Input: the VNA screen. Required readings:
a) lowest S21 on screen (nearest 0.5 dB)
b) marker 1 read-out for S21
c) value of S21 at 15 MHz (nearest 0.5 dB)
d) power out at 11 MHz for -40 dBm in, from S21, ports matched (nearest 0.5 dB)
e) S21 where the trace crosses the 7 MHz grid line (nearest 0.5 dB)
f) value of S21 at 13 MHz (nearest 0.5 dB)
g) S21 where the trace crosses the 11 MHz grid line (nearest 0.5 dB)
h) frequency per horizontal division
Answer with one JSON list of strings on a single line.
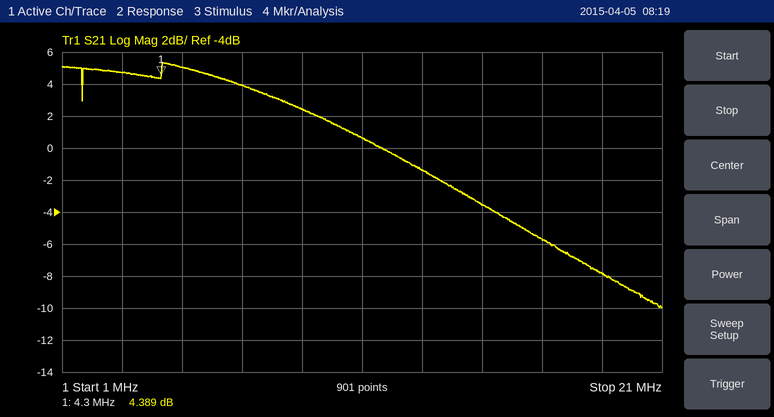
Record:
["-10.0 dB", "4.389 dB", "-3.5 dB", "-39.5 dBm", "4.0 dB", "-1.5 dB", "0.5 dB", "2 MHz"]
